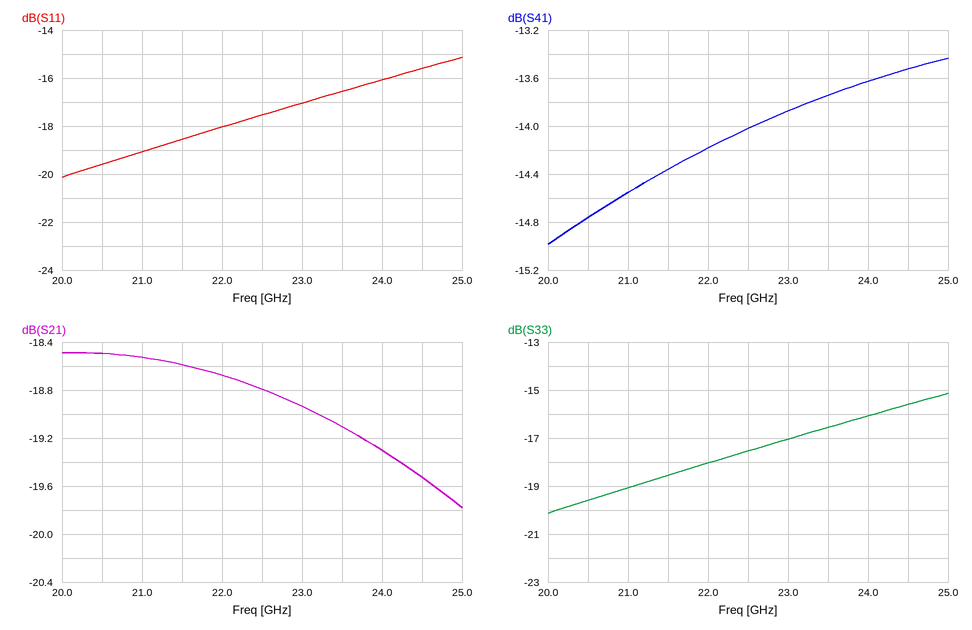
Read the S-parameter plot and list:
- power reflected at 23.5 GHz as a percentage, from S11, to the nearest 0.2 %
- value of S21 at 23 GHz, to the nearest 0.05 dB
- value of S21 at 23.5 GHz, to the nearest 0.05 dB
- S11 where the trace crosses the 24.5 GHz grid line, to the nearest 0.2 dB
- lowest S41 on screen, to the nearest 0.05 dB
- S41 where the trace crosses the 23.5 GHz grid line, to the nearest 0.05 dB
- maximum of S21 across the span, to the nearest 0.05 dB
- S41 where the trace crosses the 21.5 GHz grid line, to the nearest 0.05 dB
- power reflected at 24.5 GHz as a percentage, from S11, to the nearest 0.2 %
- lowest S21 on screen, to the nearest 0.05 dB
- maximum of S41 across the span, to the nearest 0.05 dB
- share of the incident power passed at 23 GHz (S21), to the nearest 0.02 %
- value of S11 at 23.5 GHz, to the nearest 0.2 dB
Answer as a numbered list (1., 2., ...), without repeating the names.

1. 2.2 %
2. -18.95 dB
3. -19.10 dB
4. -15.6 dB
5. -15.00 dB
6. -13.75 dB
7. -18.50 dB
8. -14.35 dB
9. 2.8 %
10. -19.80 dB
11. -13.45 dB
12. 1.28 %
13. -16.6 dB
